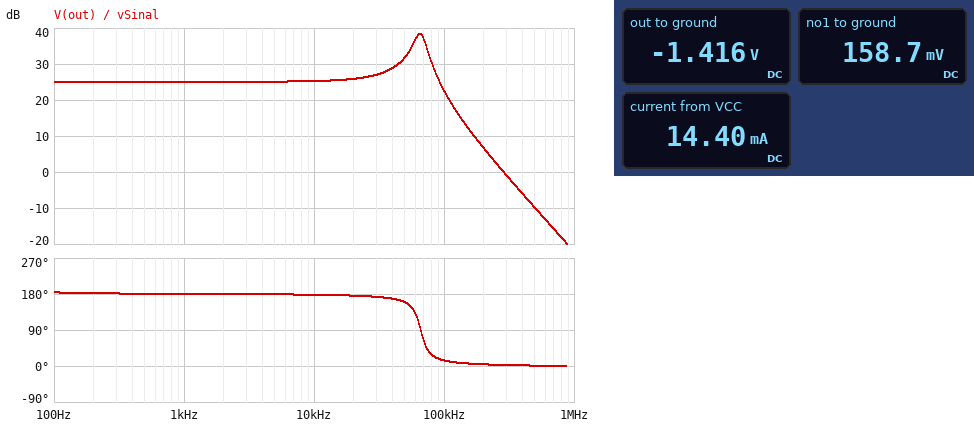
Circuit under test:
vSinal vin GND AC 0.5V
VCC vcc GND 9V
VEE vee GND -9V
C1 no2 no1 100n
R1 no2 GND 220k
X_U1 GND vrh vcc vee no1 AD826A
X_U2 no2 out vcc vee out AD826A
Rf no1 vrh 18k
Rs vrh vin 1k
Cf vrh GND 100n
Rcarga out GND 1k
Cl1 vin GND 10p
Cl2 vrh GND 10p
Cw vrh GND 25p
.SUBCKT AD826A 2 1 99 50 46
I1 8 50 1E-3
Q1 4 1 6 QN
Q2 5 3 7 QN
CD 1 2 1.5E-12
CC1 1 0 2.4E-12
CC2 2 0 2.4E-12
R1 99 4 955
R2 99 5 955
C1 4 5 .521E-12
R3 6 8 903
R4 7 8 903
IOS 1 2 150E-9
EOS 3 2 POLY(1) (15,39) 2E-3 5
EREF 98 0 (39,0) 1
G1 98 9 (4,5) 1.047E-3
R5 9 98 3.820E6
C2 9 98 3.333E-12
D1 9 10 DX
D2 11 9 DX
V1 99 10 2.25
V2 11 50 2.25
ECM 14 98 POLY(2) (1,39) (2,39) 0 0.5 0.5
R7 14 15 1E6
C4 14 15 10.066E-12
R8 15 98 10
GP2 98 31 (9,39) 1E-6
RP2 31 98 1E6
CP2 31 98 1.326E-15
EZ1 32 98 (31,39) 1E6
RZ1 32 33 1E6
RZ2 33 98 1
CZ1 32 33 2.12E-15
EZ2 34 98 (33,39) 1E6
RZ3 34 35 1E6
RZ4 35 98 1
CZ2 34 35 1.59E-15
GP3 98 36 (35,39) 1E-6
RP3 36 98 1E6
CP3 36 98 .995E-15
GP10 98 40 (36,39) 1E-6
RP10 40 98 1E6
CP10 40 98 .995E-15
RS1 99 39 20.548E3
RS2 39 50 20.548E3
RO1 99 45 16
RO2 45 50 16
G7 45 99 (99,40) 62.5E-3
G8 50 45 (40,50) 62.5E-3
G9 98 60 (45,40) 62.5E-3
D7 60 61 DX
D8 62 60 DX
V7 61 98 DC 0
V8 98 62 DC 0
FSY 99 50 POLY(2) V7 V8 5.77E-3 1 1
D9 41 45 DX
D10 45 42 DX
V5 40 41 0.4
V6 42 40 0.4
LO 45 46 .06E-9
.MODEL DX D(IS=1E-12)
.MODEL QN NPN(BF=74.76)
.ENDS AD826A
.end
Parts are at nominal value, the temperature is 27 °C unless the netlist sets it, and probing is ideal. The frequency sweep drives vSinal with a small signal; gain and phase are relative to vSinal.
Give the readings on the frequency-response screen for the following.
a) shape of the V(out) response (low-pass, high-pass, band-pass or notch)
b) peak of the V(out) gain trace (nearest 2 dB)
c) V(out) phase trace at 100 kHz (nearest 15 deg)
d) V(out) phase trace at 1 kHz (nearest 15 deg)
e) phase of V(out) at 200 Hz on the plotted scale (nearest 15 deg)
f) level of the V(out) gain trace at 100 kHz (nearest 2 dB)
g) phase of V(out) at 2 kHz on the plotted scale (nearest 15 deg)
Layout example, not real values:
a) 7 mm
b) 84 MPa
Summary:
a) low-pass
b) 38 dB
c) 15 deg
d) 180 deg
e) 180 deg
f) 22 dB
g) 180 deg
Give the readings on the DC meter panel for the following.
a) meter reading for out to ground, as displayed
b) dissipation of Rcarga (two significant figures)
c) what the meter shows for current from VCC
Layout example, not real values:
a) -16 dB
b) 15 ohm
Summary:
a) -1.416 V
b) 2.0 mW
c) 14.40 mA
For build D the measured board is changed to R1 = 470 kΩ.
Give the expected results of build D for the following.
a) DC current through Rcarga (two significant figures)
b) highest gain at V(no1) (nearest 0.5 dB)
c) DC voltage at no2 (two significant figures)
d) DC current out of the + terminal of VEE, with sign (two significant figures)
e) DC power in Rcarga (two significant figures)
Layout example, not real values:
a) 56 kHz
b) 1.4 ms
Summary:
a) 3.0 mA
b) 38.5 dB
c) -3.0 V
d) -17 mA
e) 9.2 mW
